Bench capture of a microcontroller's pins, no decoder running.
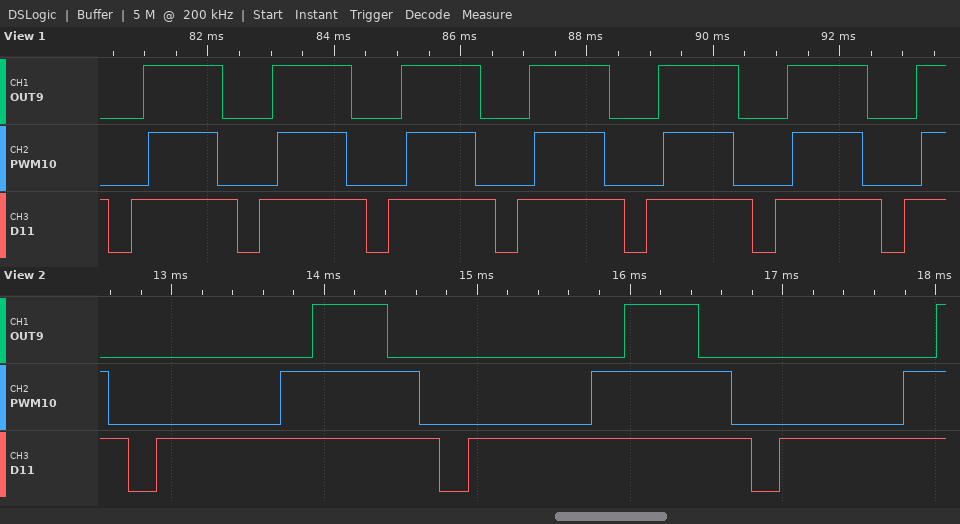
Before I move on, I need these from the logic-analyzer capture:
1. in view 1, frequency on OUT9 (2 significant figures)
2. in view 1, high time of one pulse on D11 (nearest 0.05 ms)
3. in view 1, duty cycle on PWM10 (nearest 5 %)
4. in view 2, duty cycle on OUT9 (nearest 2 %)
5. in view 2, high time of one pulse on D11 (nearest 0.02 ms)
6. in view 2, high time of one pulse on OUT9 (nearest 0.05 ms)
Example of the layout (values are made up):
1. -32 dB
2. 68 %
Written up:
1. 490 Hz
2. 1.70 ms
3. 55 %
4. 24 %
5. 1.86 ms
6. 0.50 ms
